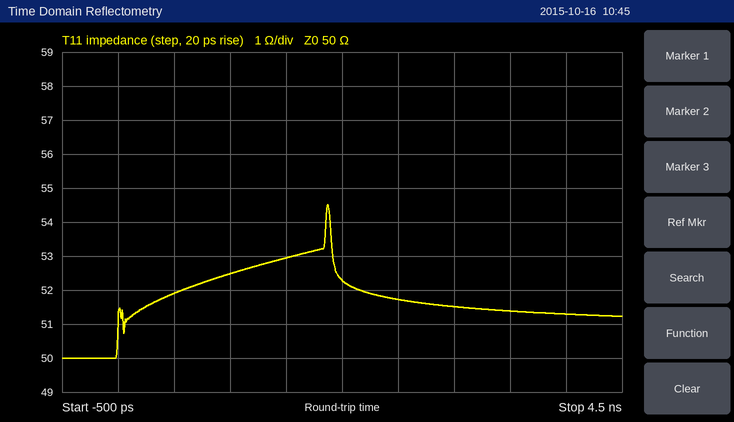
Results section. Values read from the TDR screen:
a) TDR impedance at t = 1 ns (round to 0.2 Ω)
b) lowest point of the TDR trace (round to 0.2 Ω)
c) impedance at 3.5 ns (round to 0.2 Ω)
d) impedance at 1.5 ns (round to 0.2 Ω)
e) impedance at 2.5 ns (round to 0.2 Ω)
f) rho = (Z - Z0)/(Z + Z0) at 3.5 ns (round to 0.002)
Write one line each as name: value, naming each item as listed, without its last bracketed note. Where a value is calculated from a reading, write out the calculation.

TDR impedance at t = 1 ns: 52.4 Ω
lowest point of the TDR trace: 50.0 Ω
impedance at 3.5 ns: 51.4 Ω
impedance at 1.5 ns: 53.0 Ω
impedance at 2.5 ns: 51.8 Ω
rho = (Z - Z0)/(Z + Z0) at 3.5 ns: (51.4 − 50)/(51.4 + 50) ≈ +0.014
